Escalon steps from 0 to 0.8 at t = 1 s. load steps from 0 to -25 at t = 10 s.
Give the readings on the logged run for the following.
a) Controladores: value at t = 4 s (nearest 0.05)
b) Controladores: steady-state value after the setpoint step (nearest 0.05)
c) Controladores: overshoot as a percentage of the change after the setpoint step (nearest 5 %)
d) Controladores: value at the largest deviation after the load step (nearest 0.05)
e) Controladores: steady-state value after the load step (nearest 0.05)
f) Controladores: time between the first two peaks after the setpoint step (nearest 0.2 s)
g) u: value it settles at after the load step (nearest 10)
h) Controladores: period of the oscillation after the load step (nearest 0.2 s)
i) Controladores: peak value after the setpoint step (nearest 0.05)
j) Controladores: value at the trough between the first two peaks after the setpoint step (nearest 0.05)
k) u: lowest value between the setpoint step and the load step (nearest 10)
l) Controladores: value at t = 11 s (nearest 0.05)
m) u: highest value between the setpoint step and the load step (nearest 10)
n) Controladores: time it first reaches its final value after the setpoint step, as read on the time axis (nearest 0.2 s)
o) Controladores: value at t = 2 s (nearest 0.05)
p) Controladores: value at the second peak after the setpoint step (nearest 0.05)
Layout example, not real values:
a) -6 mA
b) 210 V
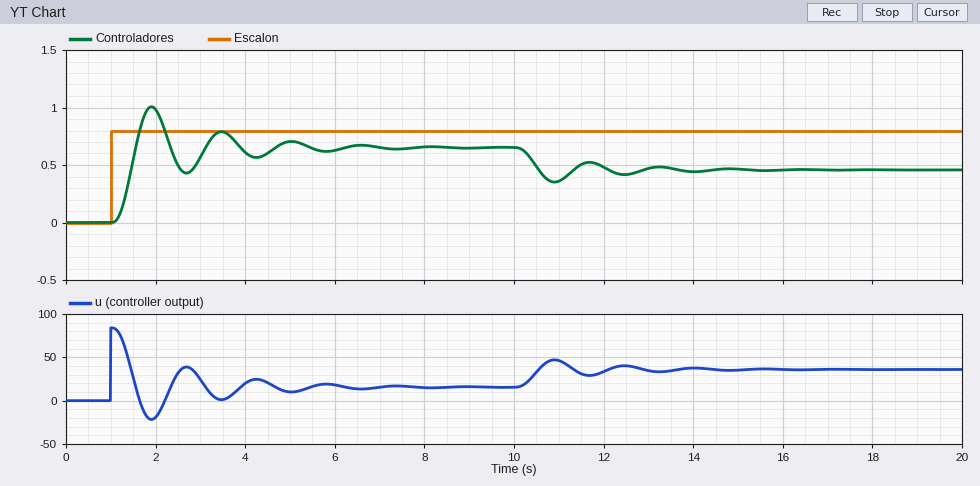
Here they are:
a) 0.60
b) 0.65
c) 55 %
d) 0.35
e) 0.45
f) 1.6 s
g) 40
h) 1.6 s
i) 1.00
j) 0.45
k) -20
l) 0.35
m) 80
n) 1.6 s
o) 1.00
p) 0.80
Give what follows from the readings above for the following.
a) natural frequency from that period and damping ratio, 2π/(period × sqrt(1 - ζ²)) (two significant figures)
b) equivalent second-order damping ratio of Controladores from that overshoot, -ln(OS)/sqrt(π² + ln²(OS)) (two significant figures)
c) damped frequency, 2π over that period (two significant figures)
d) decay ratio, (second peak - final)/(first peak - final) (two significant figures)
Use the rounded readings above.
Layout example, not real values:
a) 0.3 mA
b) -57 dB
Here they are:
a) 4.0 rad/s
b) 0.19
c) 3.9 rad/s
d) 0.43
